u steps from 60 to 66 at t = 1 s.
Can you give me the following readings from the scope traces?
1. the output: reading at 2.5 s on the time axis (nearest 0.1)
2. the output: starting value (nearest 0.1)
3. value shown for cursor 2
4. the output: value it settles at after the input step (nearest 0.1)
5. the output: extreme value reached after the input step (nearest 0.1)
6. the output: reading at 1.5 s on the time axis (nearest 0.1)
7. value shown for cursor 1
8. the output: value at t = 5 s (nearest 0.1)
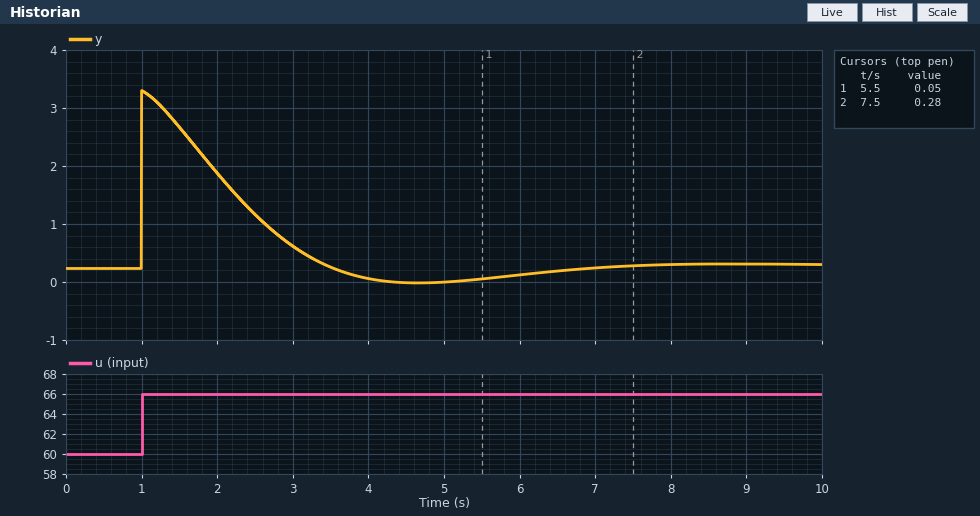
1.2
0.2
0.28
0.3
3.3
2.7
0.05
0.0
